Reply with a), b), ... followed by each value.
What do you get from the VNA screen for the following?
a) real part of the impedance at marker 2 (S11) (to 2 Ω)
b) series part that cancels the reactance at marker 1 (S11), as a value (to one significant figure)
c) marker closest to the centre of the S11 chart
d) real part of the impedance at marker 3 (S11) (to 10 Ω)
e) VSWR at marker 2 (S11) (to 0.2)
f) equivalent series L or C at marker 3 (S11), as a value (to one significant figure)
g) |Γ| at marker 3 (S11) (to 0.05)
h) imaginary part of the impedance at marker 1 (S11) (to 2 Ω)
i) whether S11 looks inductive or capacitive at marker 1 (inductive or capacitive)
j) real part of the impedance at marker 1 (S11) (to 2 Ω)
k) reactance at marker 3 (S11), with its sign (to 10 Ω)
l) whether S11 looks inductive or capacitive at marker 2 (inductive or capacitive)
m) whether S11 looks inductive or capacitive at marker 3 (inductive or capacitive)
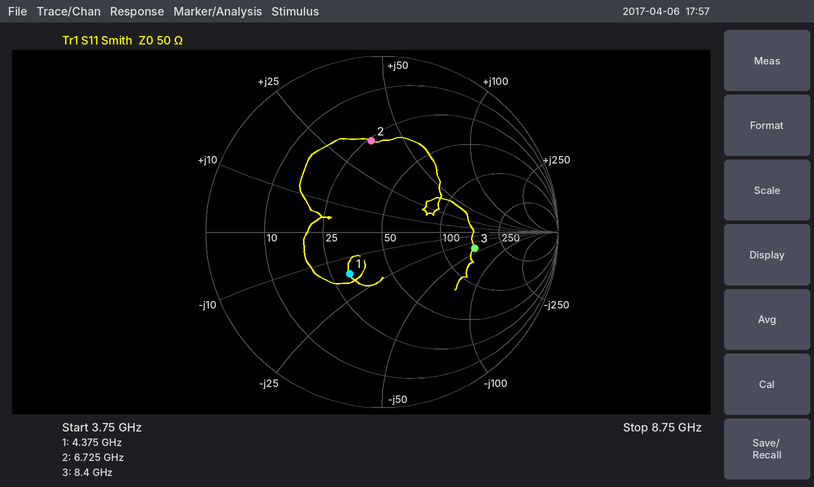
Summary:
a) 26 Ω
b) 600 pH
c) marker 1
d) 150 Ω
e) 3.2
f) 500 fF
g) 0.55
h) -16 Ω
i) capacitive
j) 32 Ω
k) -40 Ω
l) inductive
m) capacitive
